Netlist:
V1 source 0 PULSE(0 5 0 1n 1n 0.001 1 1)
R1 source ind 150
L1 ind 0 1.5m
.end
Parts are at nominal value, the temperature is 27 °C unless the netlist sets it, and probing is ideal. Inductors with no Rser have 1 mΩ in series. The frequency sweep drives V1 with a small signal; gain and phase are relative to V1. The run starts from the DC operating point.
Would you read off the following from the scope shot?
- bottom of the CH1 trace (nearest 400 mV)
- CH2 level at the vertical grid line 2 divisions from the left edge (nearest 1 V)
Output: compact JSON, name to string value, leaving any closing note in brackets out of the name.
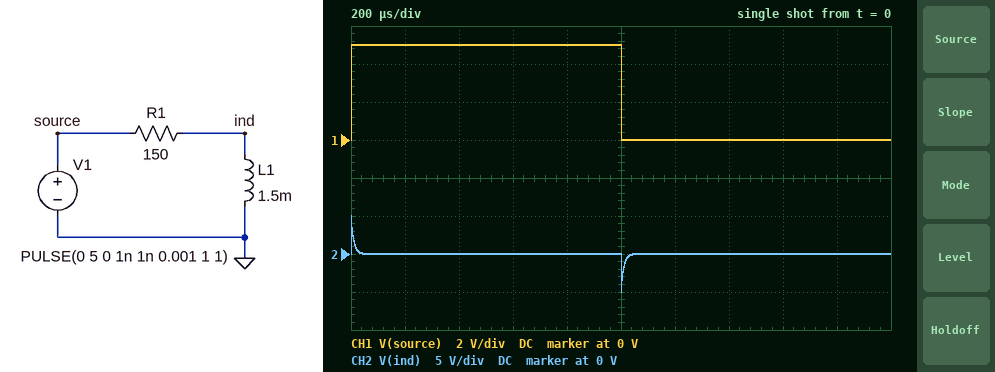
{"bottom of the CH1 trace": "0 V", "CH2 level at the vertical grid line 2 divisions from the left edge": "0 V"}
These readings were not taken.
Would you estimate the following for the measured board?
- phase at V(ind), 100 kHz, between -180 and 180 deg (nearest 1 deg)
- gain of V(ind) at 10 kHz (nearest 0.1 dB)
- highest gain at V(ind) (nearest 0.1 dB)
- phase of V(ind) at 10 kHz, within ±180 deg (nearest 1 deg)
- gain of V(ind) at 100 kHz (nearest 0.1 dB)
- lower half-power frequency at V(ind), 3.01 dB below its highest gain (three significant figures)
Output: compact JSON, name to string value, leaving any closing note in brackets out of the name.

{"phase at V(ind), 100 kHz, between -180 and 180 deg": "9 deg", "gain of V(ind) at 10 kHz": "-5.5 dB", "highest gain at V(ind)": "0 dB", "phase of V(ind) at 10 kHz, within ±180 deg": "58 deg", "gain of V(ind) at 100 kHz": "-0.1 dB", "lower half-power frequency at V(ind), 3.01 dB below its highest gain": "15.9 kHz"}
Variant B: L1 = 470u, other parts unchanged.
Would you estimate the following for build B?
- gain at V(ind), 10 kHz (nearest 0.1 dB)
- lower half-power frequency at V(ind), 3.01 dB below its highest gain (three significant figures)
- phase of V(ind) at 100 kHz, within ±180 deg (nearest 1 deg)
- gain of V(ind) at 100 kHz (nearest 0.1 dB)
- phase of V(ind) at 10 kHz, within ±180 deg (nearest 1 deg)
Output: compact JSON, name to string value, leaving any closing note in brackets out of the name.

{"gain at V(ind), 10 kHz": "-14.3 dB", "lower half-power frequency at V(ind), 3.01 dB below its highest gain": "50.8 kHz", "phase of V(ind) at 100 kHz, within ±180 deg": "27 deg", "gain of V(ind) at 100 kHz": "-1.0 dB", "phase of V(ind) at 10 kHz, within ±180 deg": "79 deg"}
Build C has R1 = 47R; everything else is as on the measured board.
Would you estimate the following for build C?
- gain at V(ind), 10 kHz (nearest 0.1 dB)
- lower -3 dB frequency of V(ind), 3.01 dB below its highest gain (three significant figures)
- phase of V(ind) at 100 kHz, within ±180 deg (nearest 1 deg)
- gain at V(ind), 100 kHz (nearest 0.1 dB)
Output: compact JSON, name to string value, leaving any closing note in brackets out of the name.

{"gain at V(ind), 10 kHz": "-1.0 dB", "lower -3 dB frequency of V(ind), 3.01 dB below its highest gain": "4.99 kHz", "phase of V(ind) at 100 kHz, within ±180 deg": "3 deg", "gain at V(ind), 100 kHz": "0 dB"}
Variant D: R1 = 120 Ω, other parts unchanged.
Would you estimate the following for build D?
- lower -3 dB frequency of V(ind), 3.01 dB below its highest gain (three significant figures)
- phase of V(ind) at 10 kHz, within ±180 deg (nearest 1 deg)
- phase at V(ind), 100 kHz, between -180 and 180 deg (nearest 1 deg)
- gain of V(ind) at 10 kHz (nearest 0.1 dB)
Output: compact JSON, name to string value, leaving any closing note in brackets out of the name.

{"lower -3 dB frequency of V(ind), 3.01 dB below its highest gain": "12.7 kHz", "phase of V(ind) at 10 kHz, within ±180 deg": "52 deg", "phase at V(ind), 100 kHz, between -180 and 180 deg": "7 deg", "gain of V(ind) at 10 kHz": "-4.2 dB"}
